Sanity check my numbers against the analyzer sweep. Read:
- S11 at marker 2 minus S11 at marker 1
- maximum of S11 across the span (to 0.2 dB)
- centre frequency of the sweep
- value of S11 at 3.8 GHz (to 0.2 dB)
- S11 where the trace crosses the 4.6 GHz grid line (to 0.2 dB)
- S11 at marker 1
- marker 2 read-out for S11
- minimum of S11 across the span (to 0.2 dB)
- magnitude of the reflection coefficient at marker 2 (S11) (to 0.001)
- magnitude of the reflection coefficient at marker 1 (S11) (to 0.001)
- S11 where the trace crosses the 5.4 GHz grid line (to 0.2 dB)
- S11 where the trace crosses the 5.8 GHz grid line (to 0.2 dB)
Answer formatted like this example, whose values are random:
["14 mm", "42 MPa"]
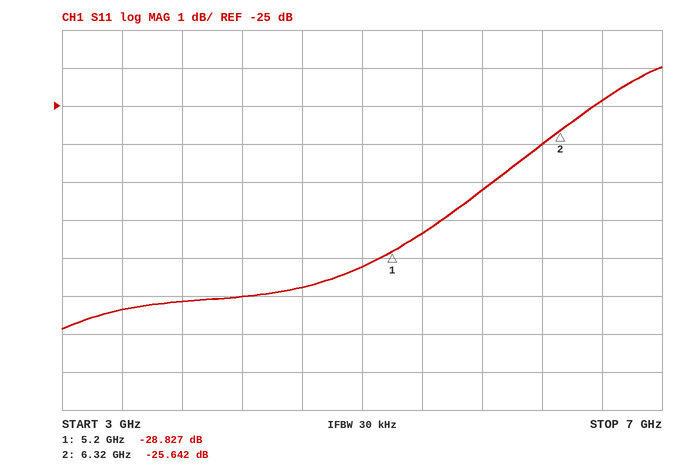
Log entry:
["3.185 dB", "-24.0 dB", "5 GHz", "-30.2 dB", "-29.8 dB", "-28.827 dB", "-25.642 dB", "-30.8 dB", "0.052", "0.036", "-28.4 dB", "-27.2 dB"]
